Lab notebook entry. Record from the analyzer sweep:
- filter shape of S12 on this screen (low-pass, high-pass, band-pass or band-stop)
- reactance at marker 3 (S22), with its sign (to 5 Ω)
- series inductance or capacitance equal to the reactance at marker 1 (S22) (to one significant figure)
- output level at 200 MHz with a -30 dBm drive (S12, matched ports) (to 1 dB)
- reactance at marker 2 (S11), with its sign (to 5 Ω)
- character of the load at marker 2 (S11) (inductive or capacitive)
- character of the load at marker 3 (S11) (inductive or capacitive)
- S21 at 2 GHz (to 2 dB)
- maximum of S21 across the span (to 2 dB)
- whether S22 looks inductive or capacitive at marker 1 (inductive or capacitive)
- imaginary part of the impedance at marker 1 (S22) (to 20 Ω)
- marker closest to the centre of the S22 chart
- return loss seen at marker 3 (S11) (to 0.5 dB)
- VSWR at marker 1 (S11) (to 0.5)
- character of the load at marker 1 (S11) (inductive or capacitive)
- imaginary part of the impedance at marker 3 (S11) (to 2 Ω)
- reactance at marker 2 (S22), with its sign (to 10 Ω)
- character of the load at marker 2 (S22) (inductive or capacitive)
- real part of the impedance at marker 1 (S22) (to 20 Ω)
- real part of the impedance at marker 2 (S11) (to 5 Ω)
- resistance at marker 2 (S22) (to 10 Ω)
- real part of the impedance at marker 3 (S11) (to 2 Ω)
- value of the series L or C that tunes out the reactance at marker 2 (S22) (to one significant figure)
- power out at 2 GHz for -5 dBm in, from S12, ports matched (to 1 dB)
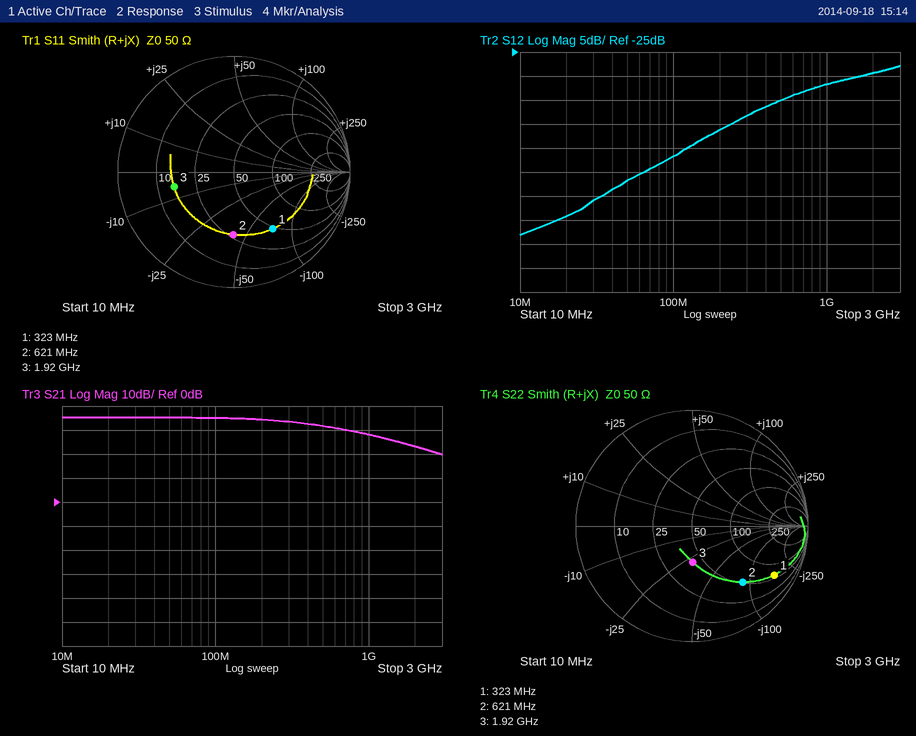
high-pass
-30 Ω
3 pF
-71 dBm
-40 Ω
capacitive
capacitive
24 dB
36 dB
capacitive
-160 Ω
marker 3
5.5 dB
4.0
capacitive
-6 Ω
-90 Ω
capacitive
60 Ω
25 Ω
50 Ω
16 Ω
20 nH
-34 dBm
